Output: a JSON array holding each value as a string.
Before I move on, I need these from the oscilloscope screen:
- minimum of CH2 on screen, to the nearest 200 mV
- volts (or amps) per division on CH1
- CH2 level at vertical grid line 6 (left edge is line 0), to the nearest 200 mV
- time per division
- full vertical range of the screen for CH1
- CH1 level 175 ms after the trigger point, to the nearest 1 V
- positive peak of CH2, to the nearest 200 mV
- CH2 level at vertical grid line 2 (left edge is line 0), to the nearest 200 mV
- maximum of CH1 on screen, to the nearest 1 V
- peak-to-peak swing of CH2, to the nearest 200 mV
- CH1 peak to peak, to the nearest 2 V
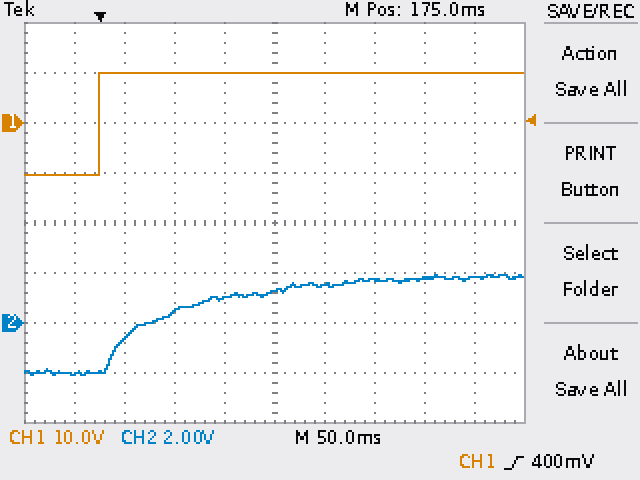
["-2.0 V", "10 V", "1.6 V", "50 ms", "80 V", "10 V", "2.0 V", "-600 mV", "10 V", "4.0 V", "20 V"]
